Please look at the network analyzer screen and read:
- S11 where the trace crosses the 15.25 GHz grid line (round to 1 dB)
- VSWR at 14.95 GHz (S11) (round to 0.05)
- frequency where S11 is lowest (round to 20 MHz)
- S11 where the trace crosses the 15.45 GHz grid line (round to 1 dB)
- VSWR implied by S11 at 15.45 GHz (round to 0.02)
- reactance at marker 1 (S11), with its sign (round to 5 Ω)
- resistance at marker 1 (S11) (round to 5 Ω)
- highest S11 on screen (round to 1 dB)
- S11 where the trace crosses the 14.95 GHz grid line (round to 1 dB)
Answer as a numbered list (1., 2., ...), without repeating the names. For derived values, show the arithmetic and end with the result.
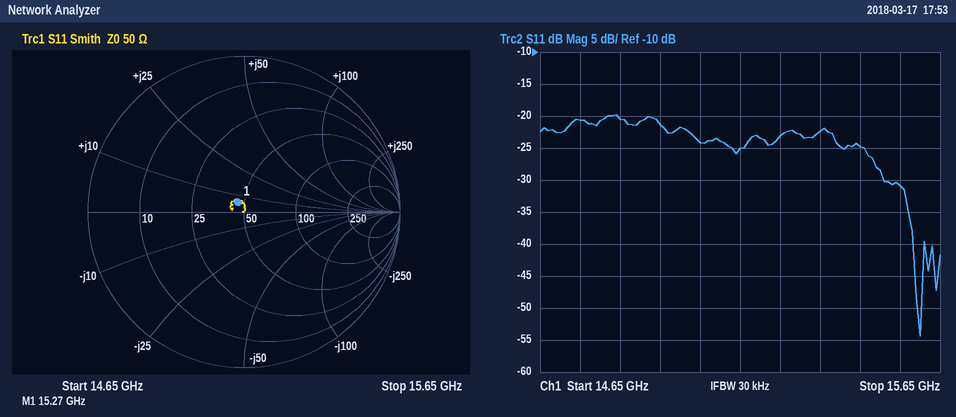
1. -23 dB
2. |Γ| = 10^(-21/20) = 0.0891; VSWR = (1 + 0.0891)/(1 − 0.0891) ≈ 1.20
3. 15.60 GHz
4. -25 dB
5. |Γ| = 10^(-25/20) = 0.0562; VSWR = (1 + 0.0562)/(1 − 0.0562) ≈ 1.12
6. +5 Ω
7. 45 Ω
8. -20 dB
9. -21 dB
